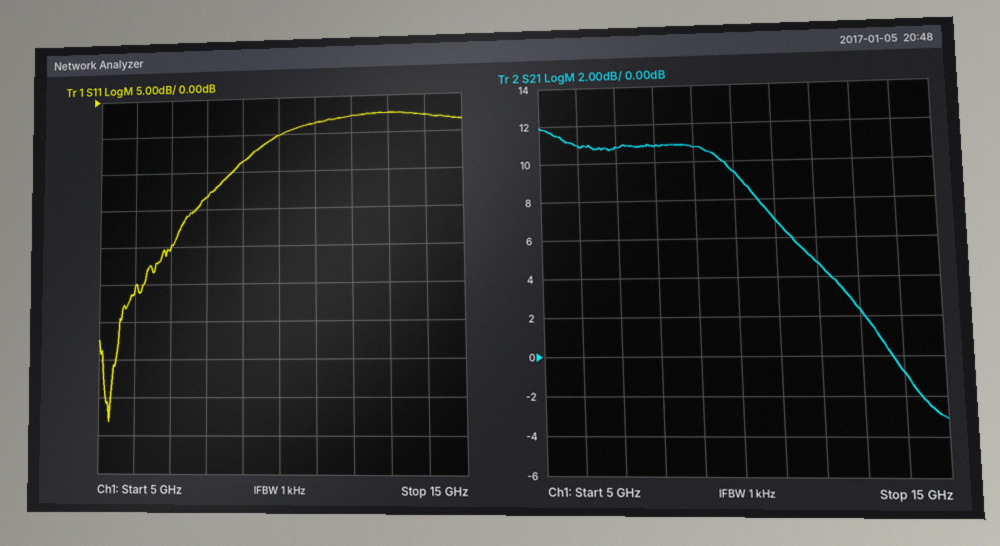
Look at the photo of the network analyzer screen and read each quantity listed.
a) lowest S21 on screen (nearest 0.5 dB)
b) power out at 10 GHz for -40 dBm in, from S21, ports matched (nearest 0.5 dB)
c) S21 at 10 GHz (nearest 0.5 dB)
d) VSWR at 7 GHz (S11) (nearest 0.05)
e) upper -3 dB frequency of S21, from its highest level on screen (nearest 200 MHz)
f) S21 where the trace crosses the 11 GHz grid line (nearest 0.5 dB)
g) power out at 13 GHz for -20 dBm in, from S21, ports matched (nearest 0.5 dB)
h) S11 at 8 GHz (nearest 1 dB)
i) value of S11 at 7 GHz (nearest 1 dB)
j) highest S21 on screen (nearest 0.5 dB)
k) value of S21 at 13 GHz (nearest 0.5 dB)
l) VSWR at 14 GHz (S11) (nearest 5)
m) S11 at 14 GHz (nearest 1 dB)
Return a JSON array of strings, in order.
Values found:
["-3.0 dB", "-30.5 dBm", "9.5 dB", "1.20", "10.2 GHz", "7.0 dB", "-17.5 dBm", "-13 dB", "-20 dB", "12.0 dB", "2.5 dB", "5", "-3 dB"]
